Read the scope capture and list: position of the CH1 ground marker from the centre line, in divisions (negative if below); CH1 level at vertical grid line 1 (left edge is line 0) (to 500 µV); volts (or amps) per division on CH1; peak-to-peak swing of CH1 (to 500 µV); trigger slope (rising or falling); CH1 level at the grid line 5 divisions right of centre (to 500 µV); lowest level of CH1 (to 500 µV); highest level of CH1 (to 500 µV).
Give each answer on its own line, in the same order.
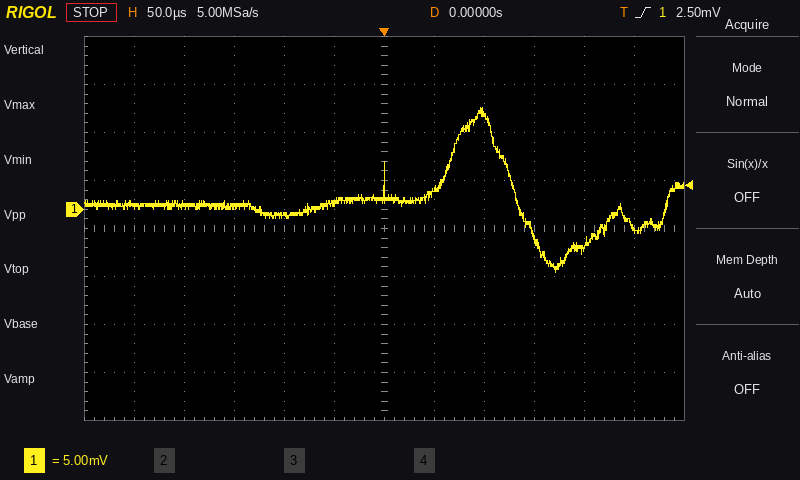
+0.4 div
500 µV
5 mV
17.0 mV
rising
-2.0 mV
-6.5 mV
10.5 mV
